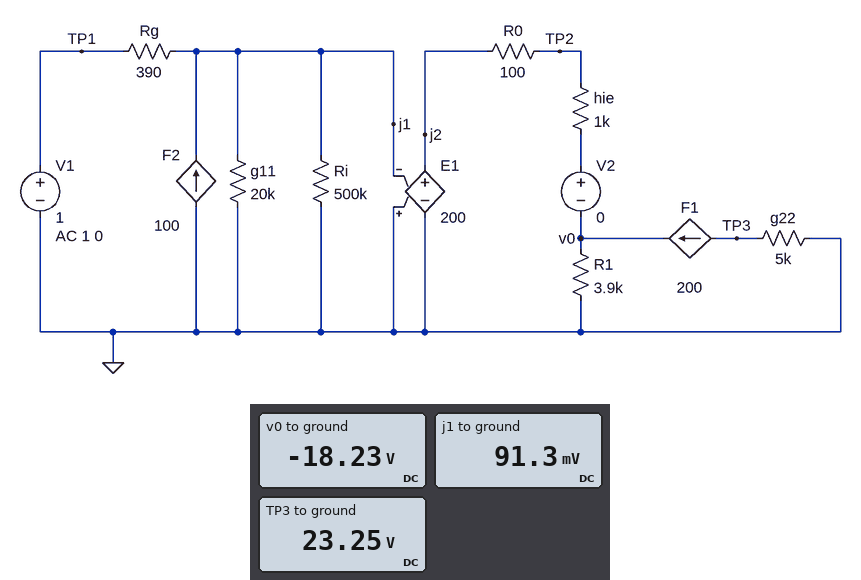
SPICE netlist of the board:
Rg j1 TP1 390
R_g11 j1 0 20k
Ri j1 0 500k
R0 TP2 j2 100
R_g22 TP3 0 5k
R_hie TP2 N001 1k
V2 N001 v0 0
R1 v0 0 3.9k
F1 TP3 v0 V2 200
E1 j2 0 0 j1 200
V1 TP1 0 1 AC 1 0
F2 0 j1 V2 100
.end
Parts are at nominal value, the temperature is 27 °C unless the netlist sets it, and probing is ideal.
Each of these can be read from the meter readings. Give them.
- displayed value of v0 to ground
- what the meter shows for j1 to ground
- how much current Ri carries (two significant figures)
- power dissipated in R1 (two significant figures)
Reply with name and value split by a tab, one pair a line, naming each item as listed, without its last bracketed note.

displayed value of v0 to ground	-18.23 V
what the meter shows for j1 to ground	91.3 mV
how much current Ri carries	180 nA
power dissipated in R1	85 mW
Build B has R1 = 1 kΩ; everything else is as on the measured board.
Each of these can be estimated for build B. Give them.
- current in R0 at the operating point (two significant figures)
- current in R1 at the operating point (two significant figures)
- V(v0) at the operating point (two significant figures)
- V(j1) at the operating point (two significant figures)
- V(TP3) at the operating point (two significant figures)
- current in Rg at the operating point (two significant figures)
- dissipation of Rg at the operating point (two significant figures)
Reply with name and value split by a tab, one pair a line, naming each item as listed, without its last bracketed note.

current in R0 at the operating point	25 µA
current in R1 at the operating point	5.0 mA
V(v0) at the operating point	-5.0 V
V(j1) at the operating point	25 mV
V(TP3) at the operating point	25 V
current in Rg at the operating point	2.5 mA
dissipation of Rg at the operating point	2.4 mW
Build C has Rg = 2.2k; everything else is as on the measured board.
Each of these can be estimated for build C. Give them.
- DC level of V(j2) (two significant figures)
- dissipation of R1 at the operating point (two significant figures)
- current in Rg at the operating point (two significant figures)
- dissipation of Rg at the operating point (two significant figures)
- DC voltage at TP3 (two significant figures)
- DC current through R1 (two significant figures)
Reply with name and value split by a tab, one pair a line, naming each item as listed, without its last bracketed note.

DC level of V(j2)	-3.5 V
dissipation of R1 at the operating point	3.1 mW
current in Rg at the operating point	450 µA
dissipation of Rg at the operating point	440 µW
DC voltage at TP3	4.5 V
DC current through R1	900 µA
